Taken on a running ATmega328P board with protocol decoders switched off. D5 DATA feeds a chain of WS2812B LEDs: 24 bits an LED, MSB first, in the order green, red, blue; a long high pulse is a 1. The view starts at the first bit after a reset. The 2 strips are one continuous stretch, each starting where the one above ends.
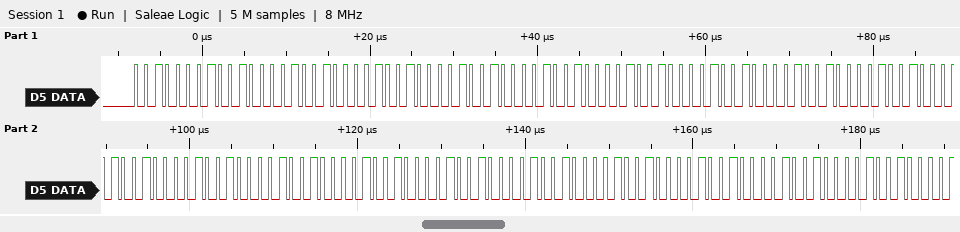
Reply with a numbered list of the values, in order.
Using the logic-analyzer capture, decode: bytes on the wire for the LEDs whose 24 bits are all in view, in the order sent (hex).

1. 21 21 21 21 21 21 21 21 21 21 21 21 21 21 21 21 21 21
